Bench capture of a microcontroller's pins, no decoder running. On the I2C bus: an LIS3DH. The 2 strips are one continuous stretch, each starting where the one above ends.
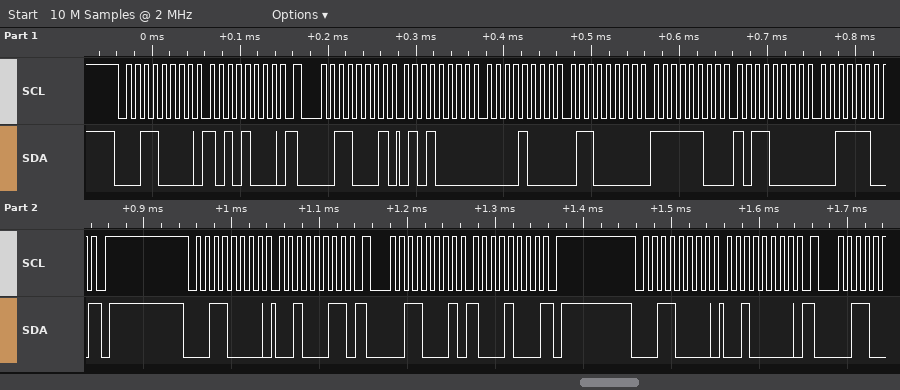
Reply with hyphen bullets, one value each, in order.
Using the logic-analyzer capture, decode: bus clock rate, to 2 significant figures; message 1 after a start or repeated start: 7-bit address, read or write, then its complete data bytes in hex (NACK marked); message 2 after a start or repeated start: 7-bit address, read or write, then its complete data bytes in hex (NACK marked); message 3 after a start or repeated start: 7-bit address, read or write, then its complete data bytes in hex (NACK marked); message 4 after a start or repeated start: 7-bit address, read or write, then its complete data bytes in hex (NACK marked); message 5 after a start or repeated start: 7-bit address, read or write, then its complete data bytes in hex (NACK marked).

- 100 kHz
- 0x18 write: A8
- 0x18 read: 50 08 60 FC B0 3C NACK
- 0x18 write: 23
- 0x18 read: 88 NACK
- 0x18 write: 20
